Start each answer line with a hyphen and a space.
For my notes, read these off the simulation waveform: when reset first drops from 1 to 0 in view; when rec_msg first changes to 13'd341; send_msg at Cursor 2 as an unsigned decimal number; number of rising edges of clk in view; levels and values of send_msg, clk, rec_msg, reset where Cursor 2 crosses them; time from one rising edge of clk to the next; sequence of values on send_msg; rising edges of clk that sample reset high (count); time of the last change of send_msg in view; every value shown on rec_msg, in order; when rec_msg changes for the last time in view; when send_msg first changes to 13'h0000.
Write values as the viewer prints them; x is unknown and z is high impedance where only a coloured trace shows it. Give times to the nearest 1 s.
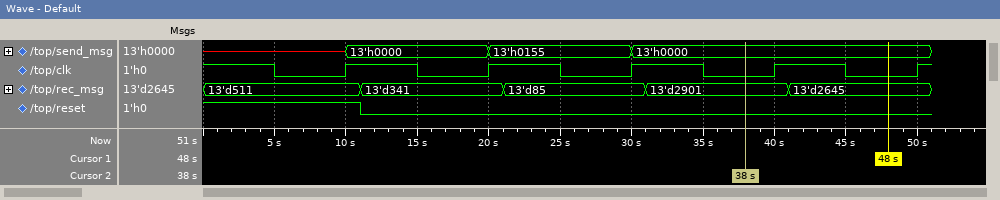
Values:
- 11 s
- 11 s
- 0
- 5
- send_msg=13'h0000, clk=0, rec_msg=13'd2901, reset=0
- 10 s
- x, 13'h0000, 13'h0155, 13'h0000
- 1
- 30 s
- 13'd511, 13'd341, 13'd85, 13'd2901, 13'd2645
- 41 s
- 10 s
